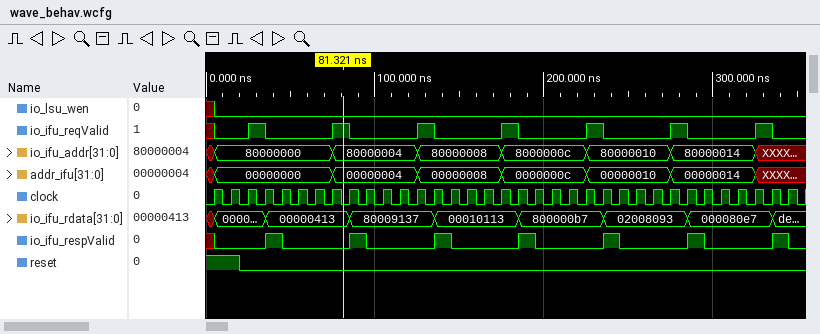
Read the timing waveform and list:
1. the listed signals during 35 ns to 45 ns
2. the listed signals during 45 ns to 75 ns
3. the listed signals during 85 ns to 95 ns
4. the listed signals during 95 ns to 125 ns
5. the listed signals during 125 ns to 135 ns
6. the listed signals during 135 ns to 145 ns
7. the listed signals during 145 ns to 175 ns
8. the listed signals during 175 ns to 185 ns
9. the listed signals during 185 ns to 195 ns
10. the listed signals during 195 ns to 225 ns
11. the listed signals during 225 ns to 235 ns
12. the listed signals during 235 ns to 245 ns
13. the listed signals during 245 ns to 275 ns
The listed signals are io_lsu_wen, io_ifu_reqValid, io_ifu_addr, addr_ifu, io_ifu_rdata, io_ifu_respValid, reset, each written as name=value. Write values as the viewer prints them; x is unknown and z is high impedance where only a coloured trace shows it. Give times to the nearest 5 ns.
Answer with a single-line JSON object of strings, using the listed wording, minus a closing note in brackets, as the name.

{"the listed signals during 35 ns to 45 ns": "io_lsu_wen=0, io_ifu_reqValid=0, io_ifu_addr=80000000, addr_ifu=00000000, io_ifu_rdata=00000413, io_ifu_respValid=1, reset=0", "the listed signals during 45 ns to 75 ns": "io_lsu_wen=0, io_ifu_reqValid=0, io_ifu_addr=80000000, addr_ifu=00000000, io_ifu_rdata=00000413, io_ifu_respValid=0, reset=0", "the listed signals during 85 ns to 95 ns": "io_lsu_wen=0, io_ifu_reqValid=0, io_ifu_addr=80000004, addr_ifu=00000004, io_ifu_rdata=80009137, io_ifu_respValid=1, reset=0", "the listed signals during 95 ns to 125 ns": "io_lsu_wen=0, io_ifu_reqValid=0, io_ifu_addr=80000004, addr_ifu=00000004, io_ifu_rdata=80009137, io_ifu_respValid=0, reset=0", "the listed signals during 125 ns to 135 ns": "io_lsu_wen=0, io_ifu_reqValid=1, io_ifu_addr=80000008, addr_ifu=00000008, io_ifu_rdata=80009137, io_ifu_respValid=0, reset=0", "the listed signals during 135 ns to 145 ns": "io_lsu_wen=0, io_ifu_reqValid=0, io_ifu_addr=80000008, addr_ifu=00000008, io_ifu_rdata=00010113, io_ifu_respValid=1, reset=0", "the listed signals during 145 ns to 175 ns": "io_lsu_wen=0, io_ifu_reqValid=0, io_ifu_addr=80000008, addr_ifu=00000008, io_ifu_rdata=00010113, io_ifu_respValid=0, reset=0", "the listed signals during 175 ns to 185 ns": "io_lsu_wen=0, io_ifu_reqValid=1, io_ifu_addr=8000000c, addr_ifu=0000000c, io_ifu_rdata=00010113, io_ifu_respValid=0, reset=0", "the listed signals during 185 ns to 195 ns": "io_lsu_wen=0, io_ifu_reqValid=0, io_ifu_addr=8000000c, addr_ifu=0000000c, io_ifu_rdata=800000b7, io_ifu_respValid=1, reset=0", "the listed signals during 195 ns to 225 ns": "io_lsu_wen=0, io_ifu_reqValid=0, io_ifu_addr=8000000c, addr_ifu=0000000c, io_ifu_rdata=800000b7, io_ifu_respValid=0, reset=0", "the listed signals during 225 ns to 235 ns": "io_lsu_wen=0, io_ifu_reqValid=1, io_ifu_addr=80000010, addr_ifu=00000010, io_ifu_rdata=800000b7, io_ifu_respValid=0, reset=0", "the listed signals during 235 ns to 245 ns": "io_lsu_wen=0, io_ifu_reqValid=0, io_ifu_addr=80000010, addr_ifu=00000010, io_ifu_rdata=02008093, io_ifu_respValid=1, reset=0", "the listed signals during 245 ns to 275 ns": "io_lsu_wen=0, io_ifu_reqValid=0, io_ifu_addr=80000010, addr_ifu=00000010, io_ifu_rdata=02008093, io_ifu_respValid=0, reset=0"}
